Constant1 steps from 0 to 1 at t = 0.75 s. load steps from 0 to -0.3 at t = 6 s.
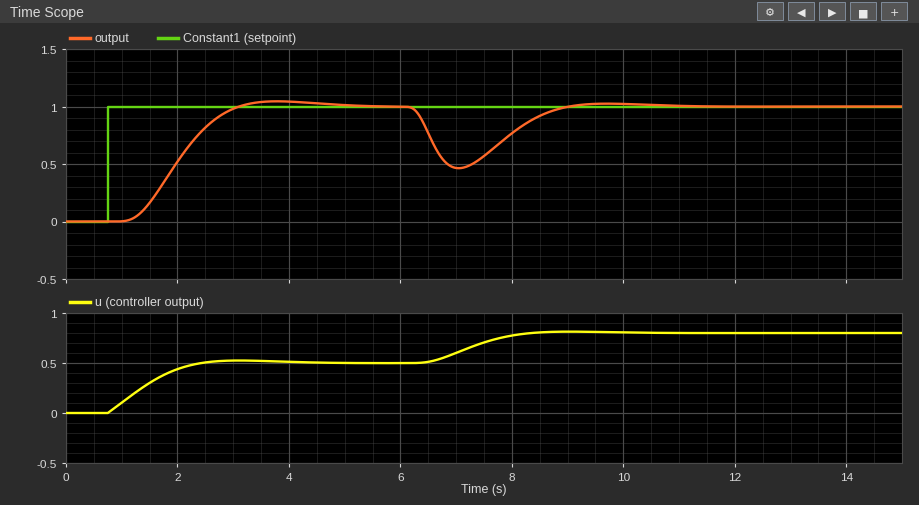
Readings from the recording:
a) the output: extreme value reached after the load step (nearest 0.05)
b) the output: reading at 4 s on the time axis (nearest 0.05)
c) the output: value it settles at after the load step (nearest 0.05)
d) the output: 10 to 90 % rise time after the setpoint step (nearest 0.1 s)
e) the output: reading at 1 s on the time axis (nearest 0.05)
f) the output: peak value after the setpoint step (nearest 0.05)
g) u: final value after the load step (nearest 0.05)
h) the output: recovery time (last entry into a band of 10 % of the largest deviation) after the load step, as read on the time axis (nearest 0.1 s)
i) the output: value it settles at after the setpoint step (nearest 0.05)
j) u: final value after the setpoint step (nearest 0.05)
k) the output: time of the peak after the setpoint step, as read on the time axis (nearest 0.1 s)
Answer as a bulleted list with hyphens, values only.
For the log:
- 0.45
- 1.05
- 1.00
- 1.3 s
- 0.00
- 1.05
- 0.80
- 8.6 s
- 1.00
- 0.50
- 3.8 s
